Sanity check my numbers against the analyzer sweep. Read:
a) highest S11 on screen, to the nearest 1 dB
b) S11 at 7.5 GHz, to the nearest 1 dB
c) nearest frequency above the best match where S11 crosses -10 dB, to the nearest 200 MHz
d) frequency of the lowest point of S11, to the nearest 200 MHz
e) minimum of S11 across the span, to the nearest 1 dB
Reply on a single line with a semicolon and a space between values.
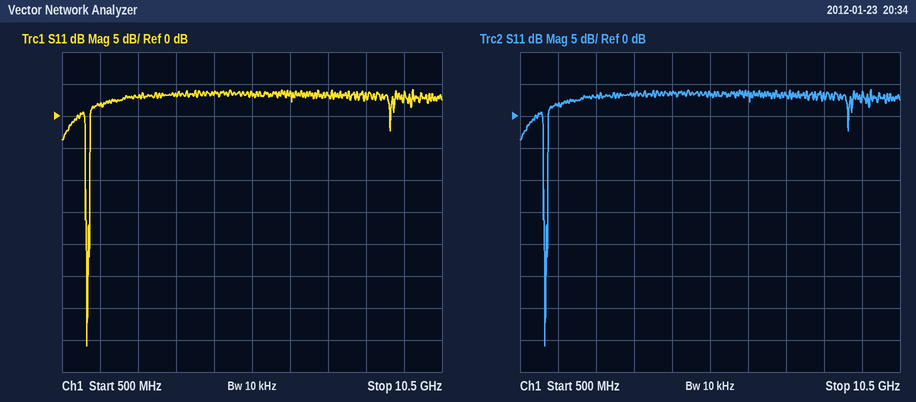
4 dB; 3 dB; 1.2 GHz; 1.2 GHz; -36 dB
